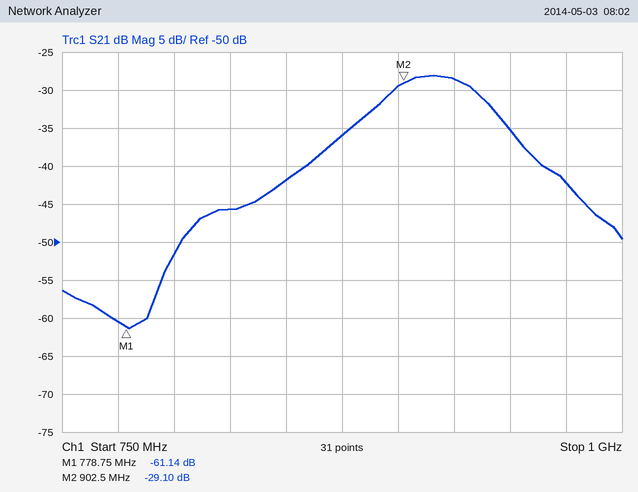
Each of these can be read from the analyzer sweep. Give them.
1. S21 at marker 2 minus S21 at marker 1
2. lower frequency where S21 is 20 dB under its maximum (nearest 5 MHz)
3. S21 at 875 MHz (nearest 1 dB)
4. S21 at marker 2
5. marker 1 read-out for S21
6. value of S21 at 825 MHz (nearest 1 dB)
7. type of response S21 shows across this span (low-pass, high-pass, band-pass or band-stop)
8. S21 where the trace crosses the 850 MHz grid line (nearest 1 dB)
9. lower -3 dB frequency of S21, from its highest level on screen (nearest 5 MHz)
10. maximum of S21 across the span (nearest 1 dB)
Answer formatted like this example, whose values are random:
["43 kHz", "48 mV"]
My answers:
["32.04 dB", "810 MHz", "-36 dB", "-29.10 dB", "-61.14 dB", "-46 dB", "band-pass", "-42 dB", "895 MHz", "-28 dB"]
